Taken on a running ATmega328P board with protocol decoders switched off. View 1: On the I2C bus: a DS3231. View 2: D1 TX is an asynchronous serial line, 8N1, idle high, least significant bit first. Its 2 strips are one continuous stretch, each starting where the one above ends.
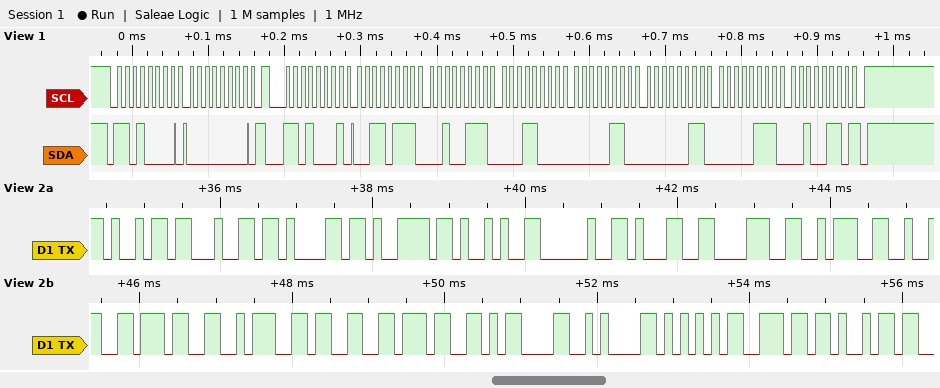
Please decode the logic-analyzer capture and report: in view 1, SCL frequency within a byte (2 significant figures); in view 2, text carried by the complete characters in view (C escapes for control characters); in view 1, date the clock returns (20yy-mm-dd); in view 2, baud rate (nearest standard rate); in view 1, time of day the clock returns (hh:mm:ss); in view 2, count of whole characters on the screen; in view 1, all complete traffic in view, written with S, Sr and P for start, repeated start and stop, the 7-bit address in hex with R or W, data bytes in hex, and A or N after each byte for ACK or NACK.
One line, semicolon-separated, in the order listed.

100 kHz; "iday) 18:27:37\r\nUni"; 2026-07-03; 9600 baud; 18:27:37; 19; S 68W A 00 A Sr 68R A 37 A 27 A 18 A 06 A 03 A 07 A 26 N P
